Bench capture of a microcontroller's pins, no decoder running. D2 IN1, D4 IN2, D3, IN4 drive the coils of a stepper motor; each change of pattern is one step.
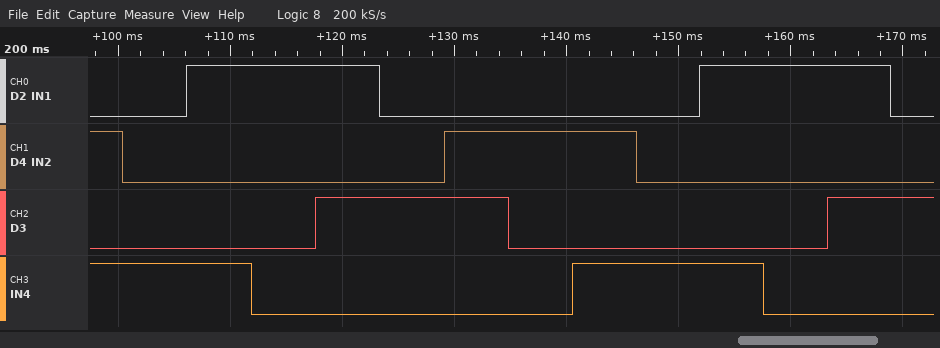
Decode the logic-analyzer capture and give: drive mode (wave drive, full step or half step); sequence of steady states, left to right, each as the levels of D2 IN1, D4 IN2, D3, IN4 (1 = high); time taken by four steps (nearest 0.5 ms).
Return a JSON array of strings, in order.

["half step", "0101 0001 1001 1000 1010 0010 0110 0100 0101 0001 1001 1000 1010 0010", "23.0 ms"]
